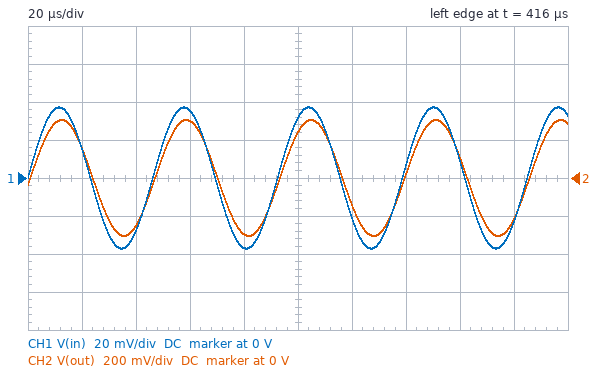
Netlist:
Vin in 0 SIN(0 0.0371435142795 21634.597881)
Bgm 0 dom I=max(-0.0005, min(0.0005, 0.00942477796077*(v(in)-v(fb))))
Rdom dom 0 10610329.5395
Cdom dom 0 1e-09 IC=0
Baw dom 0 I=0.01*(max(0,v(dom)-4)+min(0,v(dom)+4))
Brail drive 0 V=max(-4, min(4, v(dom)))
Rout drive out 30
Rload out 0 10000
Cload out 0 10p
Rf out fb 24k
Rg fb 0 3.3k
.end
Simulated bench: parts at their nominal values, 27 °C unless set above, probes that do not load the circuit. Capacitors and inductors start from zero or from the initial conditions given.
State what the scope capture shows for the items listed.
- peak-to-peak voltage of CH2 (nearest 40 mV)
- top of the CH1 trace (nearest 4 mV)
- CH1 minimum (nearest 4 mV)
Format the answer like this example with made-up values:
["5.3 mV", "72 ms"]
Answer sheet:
["600 mV", "36 mV", "-36 mV"]
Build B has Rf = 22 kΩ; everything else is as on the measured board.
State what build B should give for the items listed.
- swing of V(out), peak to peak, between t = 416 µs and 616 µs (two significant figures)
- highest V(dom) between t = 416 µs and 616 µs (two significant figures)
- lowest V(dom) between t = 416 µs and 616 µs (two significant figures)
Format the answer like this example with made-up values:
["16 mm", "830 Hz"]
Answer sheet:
["570 mV", "280 mV", "-280 mV"]
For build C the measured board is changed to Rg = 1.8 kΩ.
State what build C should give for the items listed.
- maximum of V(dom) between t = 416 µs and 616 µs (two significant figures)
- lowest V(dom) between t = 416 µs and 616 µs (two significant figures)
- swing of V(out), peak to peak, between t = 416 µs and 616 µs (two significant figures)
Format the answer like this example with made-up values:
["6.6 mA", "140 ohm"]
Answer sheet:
["520 mV", "-520 mV", "1.0 V"]
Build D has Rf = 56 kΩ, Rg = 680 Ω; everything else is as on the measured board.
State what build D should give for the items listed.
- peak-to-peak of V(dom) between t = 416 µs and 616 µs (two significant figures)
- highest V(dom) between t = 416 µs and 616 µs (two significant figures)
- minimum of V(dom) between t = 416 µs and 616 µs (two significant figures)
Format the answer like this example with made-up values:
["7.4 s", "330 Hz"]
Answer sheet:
["4.0 V", "2.0 V", "-2.0 V"]
